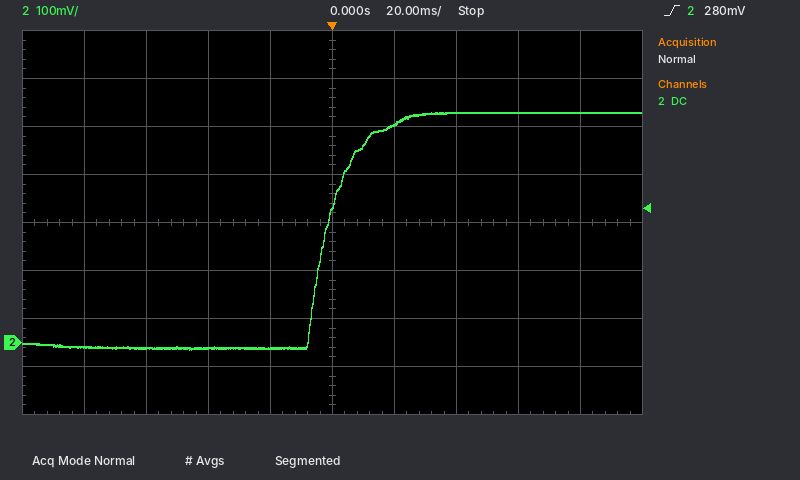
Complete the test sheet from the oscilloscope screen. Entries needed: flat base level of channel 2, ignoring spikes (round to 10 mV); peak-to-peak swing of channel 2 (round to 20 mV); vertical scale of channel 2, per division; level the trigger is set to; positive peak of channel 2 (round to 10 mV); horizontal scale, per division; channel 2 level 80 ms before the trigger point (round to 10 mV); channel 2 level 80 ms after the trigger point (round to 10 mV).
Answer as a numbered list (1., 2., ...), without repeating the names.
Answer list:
1. -10 mV
2. 500 mV
3. 100 mV
4. 280 mV
5. 480 mV
6. 20 ms
7. -10 mV
8. 480 mV
